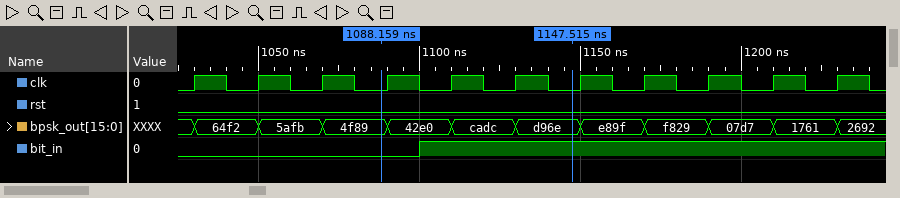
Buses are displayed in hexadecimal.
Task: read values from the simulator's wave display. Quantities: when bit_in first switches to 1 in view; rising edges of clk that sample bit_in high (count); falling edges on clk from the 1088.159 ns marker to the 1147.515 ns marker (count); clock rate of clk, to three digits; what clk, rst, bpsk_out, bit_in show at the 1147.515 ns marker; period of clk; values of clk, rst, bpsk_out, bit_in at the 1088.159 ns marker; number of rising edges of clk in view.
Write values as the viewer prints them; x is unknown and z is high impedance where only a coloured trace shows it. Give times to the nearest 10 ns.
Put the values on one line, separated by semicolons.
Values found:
1100 ns; 7; 3; 50.0 MHz; clk=0, rst=0, bpsk_out=d96e, bit_in=1; 20 ns; clk=0, rst=0, bpsk_out=4f89, bit_in=0; 11
